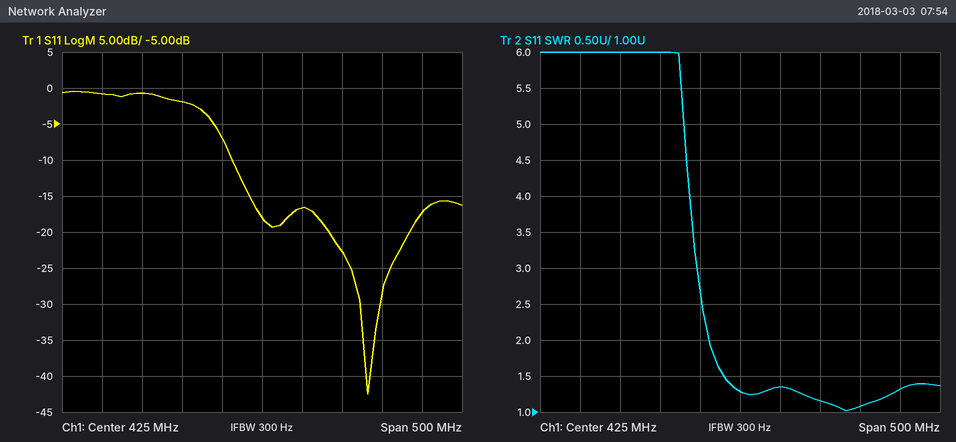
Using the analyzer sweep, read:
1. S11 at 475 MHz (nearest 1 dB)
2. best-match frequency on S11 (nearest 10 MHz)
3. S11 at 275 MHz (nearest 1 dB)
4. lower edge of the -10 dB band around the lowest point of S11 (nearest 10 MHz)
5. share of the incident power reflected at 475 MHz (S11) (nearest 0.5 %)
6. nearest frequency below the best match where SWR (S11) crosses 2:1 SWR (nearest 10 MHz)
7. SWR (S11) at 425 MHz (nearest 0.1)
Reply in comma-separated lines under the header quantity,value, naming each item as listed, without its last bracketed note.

quantity,value
S11 at 475 MHz,-17 dB
best-match frequency on S11,560 MHz
S11 at 275 MHz,-1 dB
lower edge of the -10 dB band around the lowest point of S11,390 MHz
share of the incident power reflected at 475 MHz (S11),2.0 %
nearest frequency below the best match where SWR (S11) crosses 2:1 SWR,390 MHz
SWR (S11) at 425 MHz,1.3
